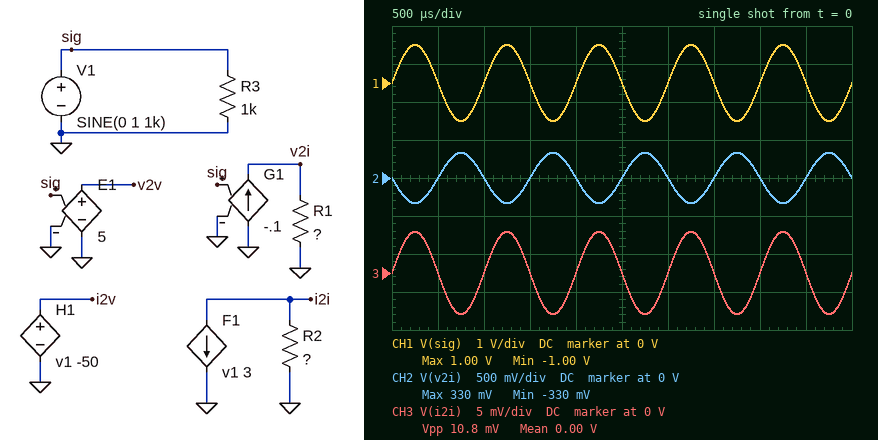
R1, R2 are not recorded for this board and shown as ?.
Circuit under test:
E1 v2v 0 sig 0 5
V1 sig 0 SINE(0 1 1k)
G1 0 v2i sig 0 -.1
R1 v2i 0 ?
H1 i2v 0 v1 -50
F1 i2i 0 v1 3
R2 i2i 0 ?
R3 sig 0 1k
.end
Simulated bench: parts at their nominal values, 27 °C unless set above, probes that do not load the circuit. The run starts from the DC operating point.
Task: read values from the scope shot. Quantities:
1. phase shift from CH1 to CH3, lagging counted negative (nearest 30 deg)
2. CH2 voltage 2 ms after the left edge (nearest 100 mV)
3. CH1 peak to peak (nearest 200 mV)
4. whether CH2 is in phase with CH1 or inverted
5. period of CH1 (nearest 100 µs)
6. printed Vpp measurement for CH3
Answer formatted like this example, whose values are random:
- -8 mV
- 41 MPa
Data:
- 0 deg
- 0 V
- 2.0 V
- inverted
- 1.0 ms
- 10.8 mV
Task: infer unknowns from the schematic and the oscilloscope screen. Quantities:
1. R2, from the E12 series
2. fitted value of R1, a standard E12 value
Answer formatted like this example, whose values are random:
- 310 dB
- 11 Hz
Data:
- 1.8 Ω
- 3.3 Ω
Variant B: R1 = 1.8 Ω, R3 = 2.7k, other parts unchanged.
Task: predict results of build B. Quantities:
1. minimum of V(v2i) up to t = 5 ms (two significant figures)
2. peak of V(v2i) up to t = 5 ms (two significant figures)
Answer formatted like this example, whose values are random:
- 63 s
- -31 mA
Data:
- -180 mV
- 180 mV
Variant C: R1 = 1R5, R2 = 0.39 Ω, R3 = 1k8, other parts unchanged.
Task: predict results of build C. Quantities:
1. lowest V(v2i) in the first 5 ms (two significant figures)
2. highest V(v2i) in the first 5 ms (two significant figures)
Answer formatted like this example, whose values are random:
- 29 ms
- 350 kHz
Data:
- -150 mV
- 150 mV
